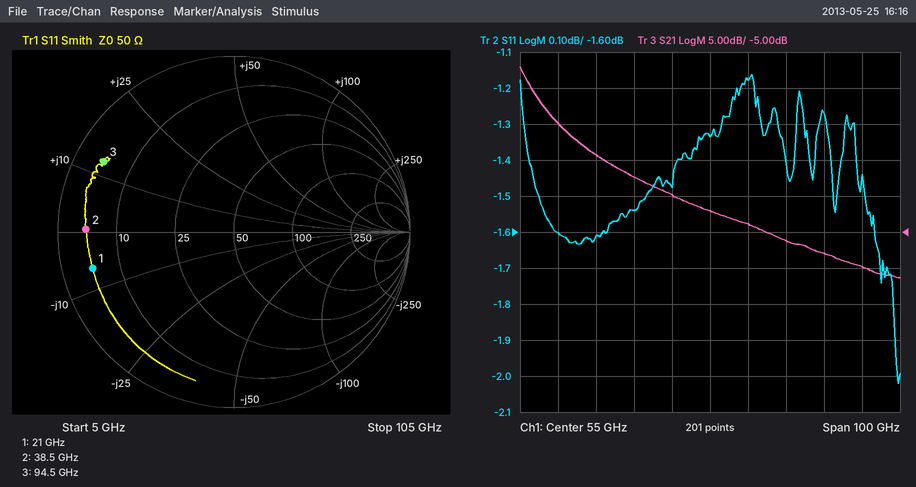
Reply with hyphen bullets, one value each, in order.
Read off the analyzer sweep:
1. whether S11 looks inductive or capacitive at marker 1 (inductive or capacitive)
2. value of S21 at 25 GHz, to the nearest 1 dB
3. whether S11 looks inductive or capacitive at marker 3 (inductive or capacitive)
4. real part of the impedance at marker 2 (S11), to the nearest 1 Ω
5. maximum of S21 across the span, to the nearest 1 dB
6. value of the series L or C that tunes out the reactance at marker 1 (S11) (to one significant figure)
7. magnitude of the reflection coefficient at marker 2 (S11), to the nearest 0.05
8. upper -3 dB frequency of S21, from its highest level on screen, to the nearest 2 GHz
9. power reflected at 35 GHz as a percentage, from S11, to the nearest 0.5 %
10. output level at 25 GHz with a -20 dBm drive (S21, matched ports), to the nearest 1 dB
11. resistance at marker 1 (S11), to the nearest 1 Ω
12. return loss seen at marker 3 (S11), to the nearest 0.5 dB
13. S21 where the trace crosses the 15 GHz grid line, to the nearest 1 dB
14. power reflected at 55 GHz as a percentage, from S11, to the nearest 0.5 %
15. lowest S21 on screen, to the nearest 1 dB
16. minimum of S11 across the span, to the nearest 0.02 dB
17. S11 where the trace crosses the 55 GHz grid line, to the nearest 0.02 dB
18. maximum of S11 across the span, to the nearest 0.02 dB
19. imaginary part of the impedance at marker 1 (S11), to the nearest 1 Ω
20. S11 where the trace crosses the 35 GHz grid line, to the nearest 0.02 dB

- capacitive
- 6 dB
- inductive
- 4 Ω
- 18 dB
- 50 pH
- 0.85
- 8 GHz
- 70.0 %
- -14 dBm
- 5 Ω
- 1.5 dB
- 10 dB
- 73.5 %
- -11 dB
- -2.02 dB
- -1.34 dB
- -1.16 dB
- -6 Ω
- -1.54 dB
